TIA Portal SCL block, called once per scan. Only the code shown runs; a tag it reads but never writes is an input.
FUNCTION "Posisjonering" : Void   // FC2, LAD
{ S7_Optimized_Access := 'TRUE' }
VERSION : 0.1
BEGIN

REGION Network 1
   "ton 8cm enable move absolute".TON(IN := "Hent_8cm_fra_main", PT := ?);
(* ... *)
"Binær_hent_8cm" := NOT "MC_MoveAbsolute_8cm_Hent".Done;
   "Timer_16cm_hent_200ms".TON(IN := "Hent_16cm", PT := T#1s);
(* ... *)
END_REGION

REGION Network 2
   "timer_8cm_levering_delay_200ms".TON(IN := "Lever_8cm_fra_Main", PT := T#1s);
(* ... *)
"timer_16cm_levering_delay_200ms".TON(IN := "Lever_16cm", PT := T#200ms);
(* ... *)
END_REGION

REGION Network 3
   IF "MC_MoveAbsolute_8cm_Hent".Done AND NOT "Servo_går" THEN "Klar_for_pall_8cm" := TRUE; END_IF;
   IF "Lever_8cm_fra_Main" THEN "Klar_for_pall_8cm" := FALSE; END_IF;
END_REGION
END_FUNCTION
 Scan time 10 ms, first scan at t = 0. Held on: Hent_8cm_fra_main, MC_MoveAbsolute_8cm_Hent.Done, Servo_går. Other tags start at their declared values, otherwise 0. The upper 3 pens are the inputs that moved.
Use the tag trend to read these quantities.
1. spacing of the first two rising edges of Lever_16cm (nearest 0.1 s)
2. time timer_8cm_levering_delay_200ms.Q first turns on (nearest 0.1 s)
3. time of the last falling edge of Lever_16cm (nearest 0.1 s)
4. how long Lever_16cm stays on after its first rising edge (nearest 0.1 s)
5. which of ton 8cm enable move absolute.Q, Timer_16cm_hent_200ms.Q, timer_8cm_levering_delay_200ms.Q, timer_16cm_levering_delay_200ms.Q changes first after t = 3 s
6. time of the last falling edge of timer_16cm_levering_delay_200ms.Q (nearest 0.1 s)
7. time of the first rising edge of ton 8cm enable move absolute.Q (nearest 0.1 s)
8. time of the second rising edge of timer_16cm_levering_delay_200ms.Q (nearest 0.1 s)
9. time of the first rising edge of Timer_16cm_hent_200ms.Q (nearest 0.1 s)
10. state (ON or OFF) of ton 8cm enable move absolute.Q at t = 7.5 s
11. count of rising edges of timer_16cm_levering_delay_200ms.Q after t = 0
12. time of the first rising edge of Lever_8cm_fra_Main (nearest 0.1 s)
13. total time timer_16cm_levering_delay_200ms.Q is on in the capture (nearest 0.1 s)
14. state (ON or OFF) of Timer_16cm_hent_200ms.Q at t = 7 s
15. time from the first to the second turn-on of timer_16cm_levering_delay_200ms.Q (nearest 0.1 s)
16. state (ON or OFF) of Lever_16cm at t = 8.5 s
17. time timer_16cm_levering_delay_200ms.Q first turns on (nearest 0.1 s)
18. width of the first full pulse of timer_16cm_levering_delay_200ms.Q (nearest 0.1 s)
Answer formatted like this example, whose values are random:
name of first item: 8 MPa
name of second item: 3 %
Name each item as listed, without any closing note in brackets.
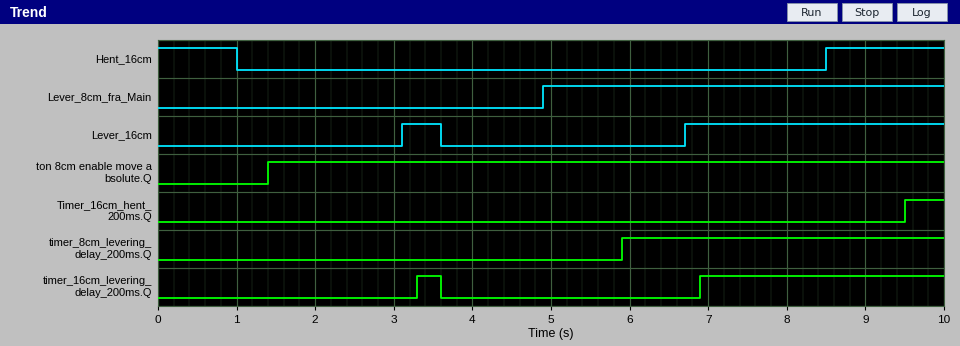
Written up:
spacing of the first two rising edges of Lever_16cm: 3.6 s
time timer_8cm_levering_delay_200ms.Q first turns on: 5.9 s
time of the last falling edge of Lever_16cm: 3.6 s
how long Lever_16cm stays on after its first rising edge: 0.5 s
which of ton 8cm enable move absolute.Q, Timer_16cm_hent_200ms.Q, timer_8cm_levering_delay_200ms.Q, timer_16cm_levering_delay_200ms.Q changes first after t = 3 s: timer_16cm_levering_delay_200ms.Q
time of the last falling edge of timer_16cm_levering_delay_200ms.Q: 3.6 s
time of the first rising edge of ton 8cm enable move absolute.Q: 1.4 s
time of the second rising edge of timer_16cm_levering_delay_200ms.Q: 6.9 s
time of the first rising edge of Timer_16cm_hent_200ms.Q: 9.5 s
state (ON or OFF) of ton 8cm enable move absolute.Q at t = 7.5 s: ON
count of rising edges of timer_16cm_levering_delay_200ms.Q after t = 0: 2
time of the first rising edge of Lever_8cm_fra_Main: 4.9 s
total time timer_16cm_levering_delay_200ms.Q is on in the capture: 3.4 s
state (ON or OFF) of Timer_16cm_hent_200ms.Q at t = 7 s: OFF
time from the first to the second turn-on of timer_16cm_levering_delay_200ms.Q: 3.6 s
state (ON or OFF) of Lever_16cm at t = 8.5 s: ON
time timer_16cm_levering_delay_200ms.Q first turns on: 3.3 s
width of the first full pulse of timer_16cm_levering_delay_200ms.Q: 0.3 s
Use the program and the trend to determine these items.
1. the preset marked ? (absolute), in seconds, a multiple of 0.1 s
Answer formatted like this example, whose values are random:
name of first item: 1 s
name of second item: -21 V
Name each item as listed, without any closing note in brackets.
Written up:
the preset marked ? (absolute), in seconds, a multiple of 0.1 s: 1.4 s
